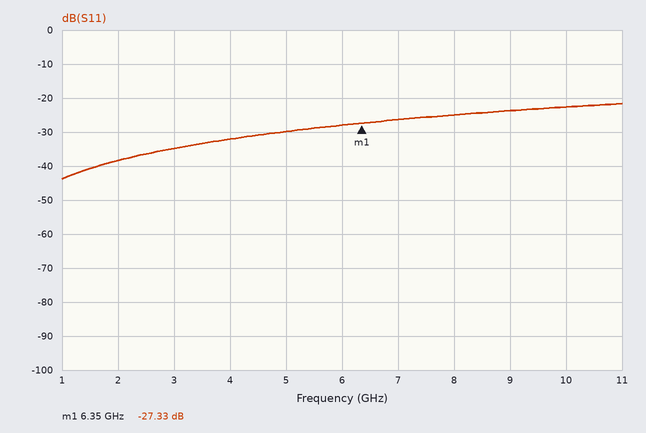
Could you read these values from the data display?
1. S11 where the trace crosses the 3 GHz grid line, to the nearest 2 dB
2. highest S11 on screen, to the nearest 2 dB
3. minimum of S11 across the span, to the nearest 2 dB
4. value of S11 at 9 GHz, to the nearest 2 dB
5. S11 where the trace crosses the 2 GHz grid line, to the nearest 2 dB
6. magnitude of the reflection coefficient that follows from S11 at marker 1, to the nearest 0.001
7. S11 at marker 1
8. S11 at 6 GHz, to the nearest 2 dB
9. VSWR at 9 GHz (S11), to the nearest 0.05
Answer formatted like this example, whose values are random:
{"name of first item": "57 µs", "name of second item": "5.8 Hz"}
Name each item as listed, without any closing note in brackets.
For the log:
{"S11 where the trace crosses the 3 GHz grid line, to the nearest 2 dB": "-34 dB", "highest S11 on screen, to the nearest 2 dB": "-22 dB", "minimum of S11 across the span, to the nearest 2 dB": "-44 dB", "value of S11 at 9 GHz, to the nearest 2 dB": "-24 dB", "S11 where the trace crosses the 2 GHz grid line, to the nearest 2 dB": "-38 dB", "magnitude of the reflection coefficient that follows from S11 at marker 1, to the nearest 0.001": "0.043", "S11 at marker 1": "-27.33 dB", "S11 at 6 GHz, to the nearest 2 dB": "-28 dB", "VSWR at 9 GHz (S11), to the nearest 0.05": "1.15"}
